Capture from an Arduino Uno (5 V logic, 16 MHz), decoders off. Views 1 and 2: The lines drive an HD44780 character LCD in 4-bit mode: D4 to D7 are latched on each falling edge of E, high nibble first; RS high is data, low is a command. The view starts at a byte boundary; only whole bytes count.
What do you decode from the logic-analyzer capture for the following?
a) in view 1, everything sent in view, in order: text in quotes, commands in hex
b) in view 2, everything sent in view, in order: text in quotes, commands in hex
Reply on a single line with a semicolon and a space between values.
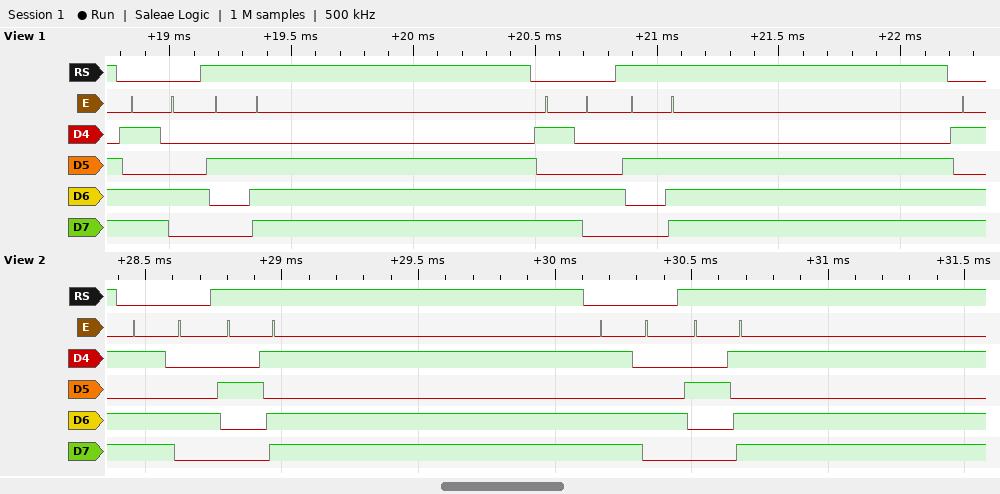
0xD4 "." 0xD4 "."; 0xD4 "-" 0xD4 "-"
